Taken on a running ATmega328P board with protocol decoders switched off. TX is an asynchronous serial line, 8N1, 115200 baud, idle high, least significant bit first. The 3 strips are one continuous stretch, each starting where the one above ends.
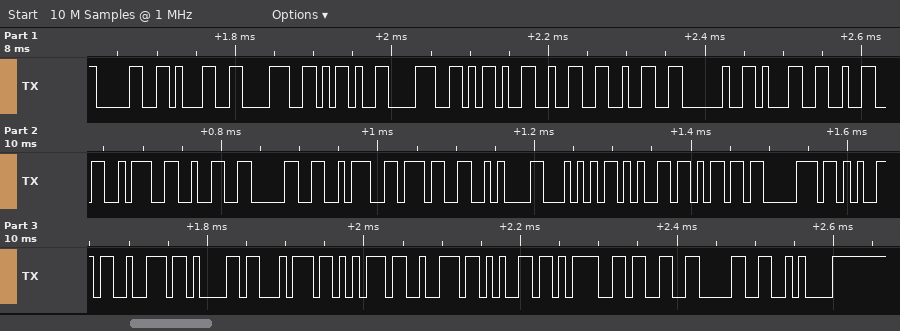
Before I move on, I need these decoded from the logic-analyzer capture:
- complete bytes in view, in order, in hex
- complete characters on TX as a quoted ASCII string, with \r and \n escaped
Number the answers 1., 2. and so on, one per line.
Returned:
1. 30 31 38 2D 38 2D 32 32 20 31 32 3A 32 30 3A 37 0A 54 65 6D 70 65 72 61 74 75 72 65 3D 33 30 0A
2. "018-8-22 12:20:7\nTemperature=30\n"
